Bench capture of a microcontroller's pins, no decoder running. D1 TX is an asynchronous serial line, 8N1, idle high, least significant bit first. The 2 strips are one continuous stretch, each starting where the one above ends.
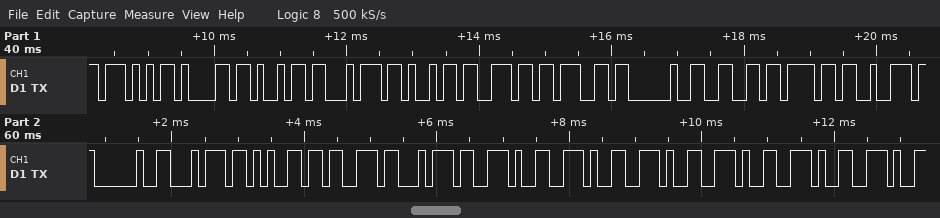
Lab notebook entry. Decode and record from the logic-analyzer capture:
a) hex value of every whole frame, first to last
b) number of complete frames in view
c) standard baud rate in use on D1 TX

57 61 69 74 69 6E 67 20 66 6F 72 20 74 65 73 74 2E 2E 2E 2E 2E 2E
22
9600 baud
